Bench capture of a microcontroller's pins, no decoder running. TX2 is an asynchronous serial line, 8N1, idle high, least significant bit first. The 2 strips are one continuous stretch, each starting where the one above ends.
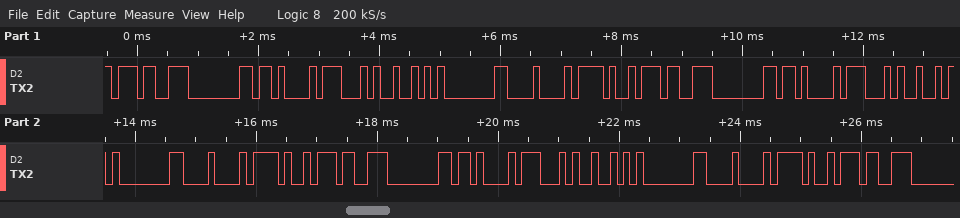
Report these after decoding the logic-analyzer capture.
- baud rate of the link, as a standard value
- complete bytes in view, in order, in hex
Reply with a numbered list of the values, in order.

1. 9600 baud
2. 37 80 0B 47 52 80 08 2F 37 80 0B 47 52 80 08 2F 37 80 0B 47 52 80 08 2F 37
